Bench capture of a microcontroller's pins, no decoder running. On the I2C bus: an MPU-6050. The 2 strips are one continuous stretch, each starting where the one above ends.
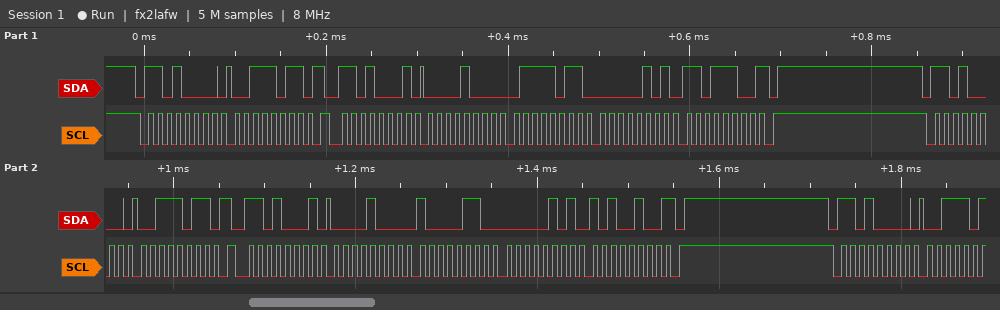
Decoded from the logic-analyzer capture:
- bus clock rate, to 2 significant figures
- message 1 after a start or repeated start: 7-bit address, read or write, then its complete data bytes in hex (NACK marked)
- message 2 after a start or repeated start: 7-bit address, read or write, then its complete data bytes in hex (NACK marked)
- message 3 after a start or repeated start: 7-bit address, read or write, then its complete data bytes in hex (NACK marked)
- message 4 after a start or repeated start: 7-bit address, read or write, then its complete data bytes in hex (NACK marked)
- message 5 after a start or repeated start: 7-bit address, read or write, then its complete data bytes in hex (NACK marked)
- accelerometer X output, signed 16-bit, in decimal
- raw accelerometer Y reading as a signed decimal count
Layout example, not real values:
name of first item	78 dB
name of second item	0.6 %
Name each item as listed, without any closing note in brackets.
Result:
bus clock rate, to 2 significant figures	100 kHz
message 1 after a start or repeated start: 7-bit address, read or write, then its complete data bytes in hex	0x68 write: 3B
message 2 after a start or repeated start: 7-bit address, read or write, then its complete data bytes in hex	0x68 read: 08 7B 05 DC NACK
message 3 after a start or repeated start: 7-bit address, read or write, then its complete data bytes in hex	0x68 write: 3B
message 4 after a start or repeated start: 7-bit address, read or write, then its complete data bytes in hex	0x68 read: 08 86 05 A4 NACK
message 5 after a start or repeated start: 7-bit address, read or write, then its complete data bytes in hex	0x68 write
accelerometer X output, signed 16-bit, in decimal	2171
raw accelerometer Y reading as a signed decimal count	1500
